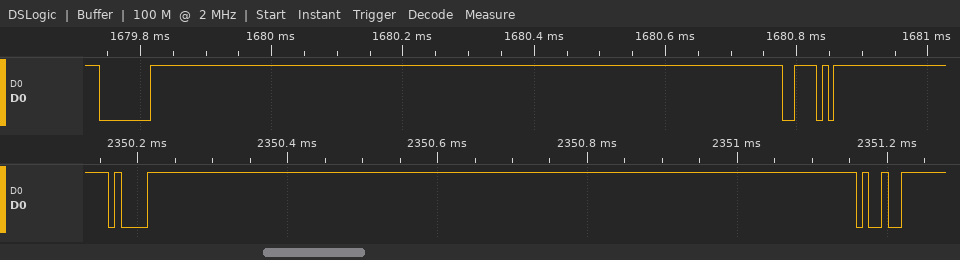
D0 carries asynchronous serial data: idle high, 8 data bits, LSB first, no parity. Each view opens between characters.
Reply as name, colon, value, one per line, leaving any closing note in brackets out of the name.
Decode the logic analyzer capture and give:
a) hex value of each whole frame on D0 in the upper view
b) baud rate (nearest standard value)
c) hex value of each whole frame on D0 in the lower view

hex value of each whole frame on D0 in the upper view: 00, 5E
baud rate: 115200 baud
hex value of each whole frame on D0 in the lower view: E1, C9
